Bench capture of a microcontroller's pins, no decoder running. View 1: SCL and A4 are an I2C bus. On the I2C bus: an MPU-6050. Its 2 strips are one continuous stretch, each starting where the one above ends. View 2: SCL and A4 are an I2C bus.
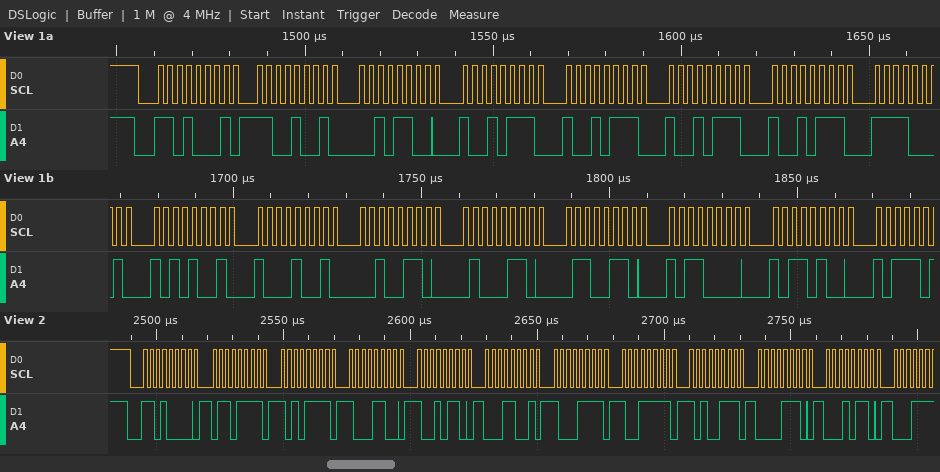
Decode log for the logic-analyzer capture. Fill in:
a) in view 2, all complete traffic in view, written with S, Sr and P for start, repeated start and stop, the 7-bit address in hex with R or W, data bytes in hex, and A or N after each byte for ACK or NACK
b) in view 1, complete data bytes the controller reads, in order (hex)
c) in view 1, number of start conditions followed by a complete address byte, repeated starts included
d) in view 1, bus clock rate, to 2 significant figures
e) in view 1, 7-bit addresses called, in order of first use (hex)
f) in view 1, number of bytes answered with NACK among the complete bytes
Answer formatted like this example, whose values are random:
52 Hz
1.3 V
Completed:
S 68W A 6F A AF A 8C A 96 A 19 A 8F A 9F A A7 A 0E A 16 A
C9 2C 97 97 97 97 F1 A9 89 26 46 66 B0 B4
1
400 kHz
0x68
0
